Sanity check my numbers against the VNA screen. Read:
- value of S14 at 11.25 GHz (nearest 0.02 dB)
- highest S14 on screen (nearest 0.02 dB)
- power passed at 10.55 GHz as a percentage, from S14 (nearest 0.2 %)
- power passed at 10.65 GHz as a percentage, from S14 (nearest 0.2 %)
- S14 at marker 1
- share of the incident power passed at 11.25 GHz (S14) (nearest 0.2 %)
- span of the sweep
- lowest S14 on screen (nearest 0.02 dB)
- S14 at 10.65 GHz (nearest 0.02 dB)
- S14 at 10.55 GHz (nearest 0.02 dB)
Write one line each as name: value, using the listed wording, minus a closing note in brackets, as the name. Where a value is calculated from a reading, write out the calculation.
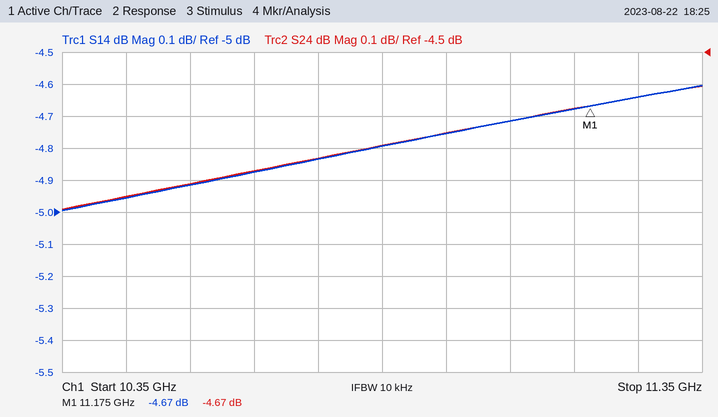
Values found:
value of S14 at 11.25 GHz: -4.64 dB
highest S14 on screen: -4.60 dB
power passed at 10.55 GHz as a percentage, from S14: 10^(-4.92/10) ≈ 32.2 %
power passed at 10.65 GHz as a percentage, from S14: 10^(-4.88/10) ≈ 32.5 %, so 32.6 % to the nearest 0.2 %
S14 at marker 1: -4.67 dB
share of the incident power passed at 11.25 GHz (S14): 10^(-4.64/10) ≈ 34.4 %
span of the sweep: 1 GHz
lowest S14 on screen: -5.00 dB
S14 at 10.65 GHz: -4.88 dB
S14 at 10.55 GHz: -4.92 dB
